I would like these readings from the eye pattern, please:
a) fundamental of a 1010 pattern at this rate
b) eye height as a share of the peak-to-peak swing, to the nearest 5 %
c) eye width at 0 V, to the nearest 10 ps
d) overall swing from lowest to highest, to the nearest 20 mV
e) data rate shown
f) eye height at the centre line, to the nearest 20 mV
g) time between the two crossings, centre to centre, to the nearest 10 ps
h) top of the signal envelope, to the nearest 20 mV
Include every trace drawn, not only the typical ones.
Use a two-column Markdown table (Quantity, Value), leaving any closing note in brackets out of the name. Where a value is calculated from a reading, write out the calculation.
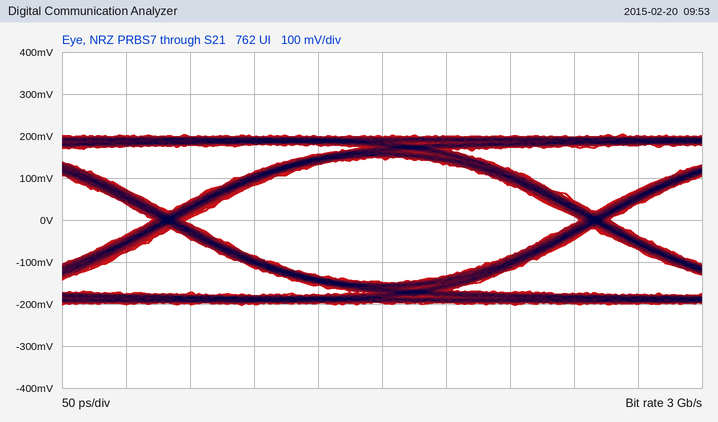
| Quantity | Value |
|---|---|
| fundamental of a 1010 pattern at this rate | 1.5 GHz |
| eye height as a share of the peak-to-peak swing, to the nearest 5 % | 300 mV / 400 mV ≈ 75 % |
| eye width at 0 V, to the nearest 10 ps | 310 ps |
| overall swing from lowest to highest, to the nearest 20 mV | 400 mV |
| data rate shown | 3 Gb/s |
| eye height at the centre line, to the nearest 20 mV | 300 mV |
| time between the two crossings, centre to centre, to the nearest 10 ps | 330 ps |
| top of the signal envelope, to the nearest 20 mV | 200 mV |
